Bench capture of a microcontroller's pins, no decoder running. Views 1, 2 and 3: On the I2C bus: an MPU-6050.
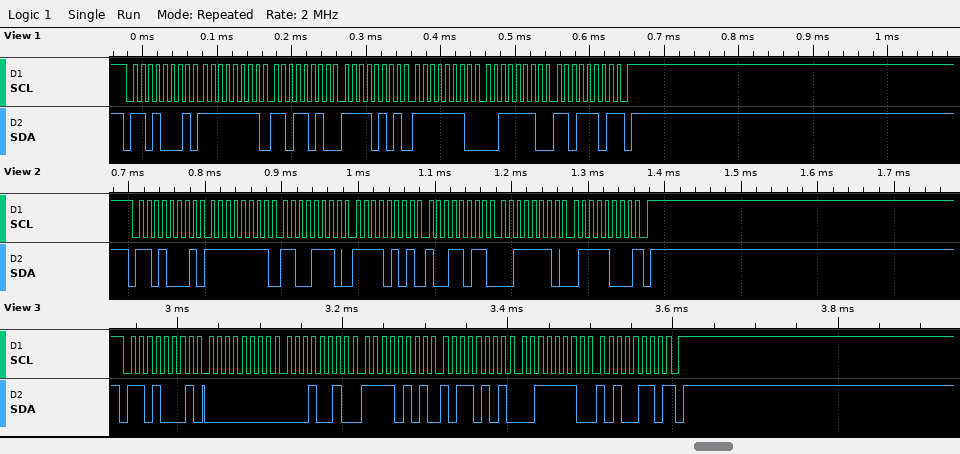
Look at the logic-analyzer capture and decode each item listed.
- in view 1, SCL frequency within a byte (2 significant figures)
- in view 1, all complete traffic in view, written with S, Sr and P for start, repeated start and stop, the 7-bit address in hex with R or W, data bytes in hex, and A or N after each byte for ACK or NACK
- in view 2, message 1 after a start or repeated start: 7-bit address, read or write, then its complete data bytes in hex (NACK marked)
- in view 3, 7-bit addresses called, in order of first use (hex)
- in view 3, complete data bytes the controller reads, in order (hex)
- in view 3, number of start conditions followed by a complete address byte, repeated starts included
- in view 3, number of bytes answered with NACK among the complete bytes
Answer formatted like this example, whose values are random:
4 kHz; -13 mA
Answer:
100 kHz; S 68R A FF A DA A F5 A FE A 3E A DD N P; 0x68 read: FF CE F5 9B 3E 78 NACK; 0x68; 00 12 F5 B5 3E A6; 1; 1
